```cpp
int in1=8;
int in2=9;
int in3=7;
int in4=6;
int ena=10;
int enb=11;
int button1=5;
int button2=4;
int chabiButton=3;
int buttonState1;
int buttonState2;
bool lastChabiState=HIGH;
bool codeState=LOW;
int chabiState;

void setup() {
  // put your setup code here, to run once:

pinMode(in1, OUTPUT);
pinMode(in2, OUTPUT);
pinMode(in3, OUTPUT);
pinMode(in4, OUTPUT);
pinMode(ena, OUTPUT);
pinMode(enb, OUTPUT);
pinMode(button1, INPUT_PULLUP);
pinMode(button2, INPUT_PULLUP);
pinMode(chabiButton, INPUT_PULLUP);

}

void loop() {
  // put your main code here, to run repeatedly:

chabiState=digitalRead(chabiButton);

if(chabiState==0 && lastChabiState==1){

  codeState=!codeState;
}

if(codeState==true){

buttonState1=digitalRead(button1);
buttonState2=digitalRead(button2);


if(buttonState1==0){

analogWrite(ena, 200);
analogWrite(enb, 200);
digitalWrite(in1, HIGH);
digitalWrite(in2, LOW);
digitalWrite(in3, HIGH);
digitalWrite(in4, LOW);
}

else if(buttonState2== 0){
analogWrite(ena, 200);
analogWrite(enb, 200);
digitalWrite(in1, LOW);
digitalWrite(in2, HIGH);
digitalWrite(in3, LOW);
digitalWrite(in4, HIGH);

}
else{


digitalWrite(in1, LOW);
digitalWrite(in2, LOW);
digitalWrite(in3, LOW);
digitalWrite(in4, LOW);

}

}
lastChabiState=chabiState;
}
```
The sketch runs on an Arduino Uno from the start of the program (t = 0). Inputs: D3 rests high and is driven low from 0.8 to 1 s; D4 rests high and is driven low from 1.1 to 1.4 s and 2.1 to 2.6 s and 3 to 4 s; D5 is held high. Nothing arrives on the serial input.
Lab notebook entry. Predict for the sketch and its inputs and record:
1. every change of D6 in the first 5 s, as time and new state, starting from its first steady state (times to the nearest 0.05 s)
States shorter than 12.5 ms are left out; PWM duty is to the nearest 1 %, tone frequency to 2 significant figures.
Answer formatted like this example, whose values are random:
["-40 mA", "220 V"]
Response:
["0 s low; 1.1 s high; 1.4 s low; 2.1 s high; 2.6 s low; 3 s high; 4 s low"]
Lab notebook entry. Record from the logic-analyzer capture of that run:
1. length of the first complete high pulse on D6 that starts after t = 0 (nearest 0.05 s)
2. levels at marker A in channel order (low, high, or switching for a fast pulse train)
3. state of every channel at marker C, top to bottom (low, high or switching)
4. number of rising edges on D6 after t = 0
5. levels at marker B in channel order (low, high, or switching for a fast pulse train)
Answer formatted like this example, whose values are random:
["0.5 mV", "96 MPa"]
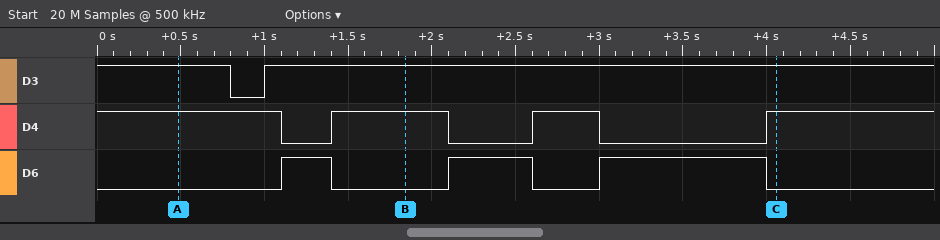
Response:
["0.30 s", "D3 high, D4 high, D6 low", "D3 high, D4 high, D6 low", "3", "D3 high, D4 high, D6 low"]
